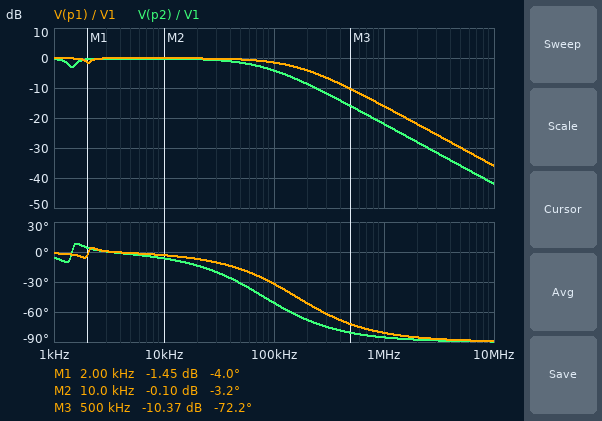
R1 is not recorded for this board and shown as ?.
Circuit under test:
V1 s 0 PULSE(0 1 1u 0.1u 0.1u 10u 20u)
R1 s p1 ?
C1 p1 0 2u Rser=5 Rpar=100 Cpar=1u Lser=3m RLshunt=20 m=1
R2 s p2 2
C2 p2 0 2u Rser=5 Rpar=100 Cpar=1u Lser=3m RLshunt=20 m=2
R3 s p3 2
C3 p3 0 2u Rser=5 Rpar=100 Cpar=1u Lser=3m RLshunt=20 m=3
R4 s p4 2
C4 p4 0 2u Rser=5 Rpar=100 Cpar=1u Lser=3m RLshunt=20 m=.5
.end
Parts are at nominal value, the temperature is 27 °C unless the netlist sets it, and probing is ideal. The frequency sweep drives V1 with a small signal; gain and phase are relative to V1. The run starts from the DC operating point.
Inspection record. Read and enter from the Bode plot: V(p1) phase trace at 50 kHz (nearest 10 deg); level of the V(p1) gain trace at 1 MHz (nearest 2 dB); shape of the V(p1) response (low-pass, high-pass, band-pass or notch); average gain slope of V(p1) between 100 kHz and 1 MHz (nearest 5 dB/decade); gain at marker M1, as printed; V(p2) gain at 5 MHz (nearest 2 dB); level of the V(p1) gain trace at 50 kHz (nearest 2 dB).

-20 deg
-16 dB
low-pass
-15 dB/decade
-1.45 dB
-36 dB
0 dB
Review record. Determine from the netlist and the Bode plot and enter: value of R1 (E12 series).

1 Ω
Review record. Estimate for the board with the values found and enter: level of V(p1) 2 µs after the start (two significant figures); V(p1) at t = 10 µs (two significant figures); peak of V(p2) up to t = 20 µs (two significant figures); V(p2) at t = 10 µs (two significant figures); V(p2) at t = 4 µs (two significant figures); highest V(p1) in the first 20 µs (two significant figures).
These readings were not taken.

610 mV
990 mV
970 mV
970 mV
760 mV
990 mV
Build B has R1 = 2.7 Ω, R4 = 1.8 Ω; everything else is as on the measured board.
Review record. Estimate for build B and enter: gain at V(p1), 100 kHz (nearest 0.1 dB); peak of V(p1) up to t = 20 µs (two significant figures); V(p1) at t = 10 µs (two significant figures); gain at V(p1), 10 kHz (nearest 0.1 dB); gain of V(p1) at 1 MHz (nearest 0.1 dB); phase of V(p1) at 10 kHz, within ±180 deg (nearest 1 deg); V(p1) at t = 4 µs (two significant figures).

-5.9 dB
950 mV
940 mV
-0.3 dB
-24.6 dB
-9 deg
660 mV
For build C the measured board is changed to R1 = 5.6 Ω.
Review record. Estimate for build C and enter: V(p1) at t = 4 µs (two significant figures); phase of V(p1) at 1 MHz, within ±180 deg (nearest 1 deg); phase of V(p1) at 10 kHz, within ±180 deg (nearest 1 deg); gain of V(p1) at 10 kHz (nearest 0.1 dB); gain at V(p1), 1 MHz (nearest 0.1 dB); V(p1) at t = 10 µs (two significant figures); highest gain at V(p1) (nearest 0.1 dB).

400 mV
-88 deg
-17 deg
-0.9 dB
-30.9 dB
770 mV
-0.5 dB
